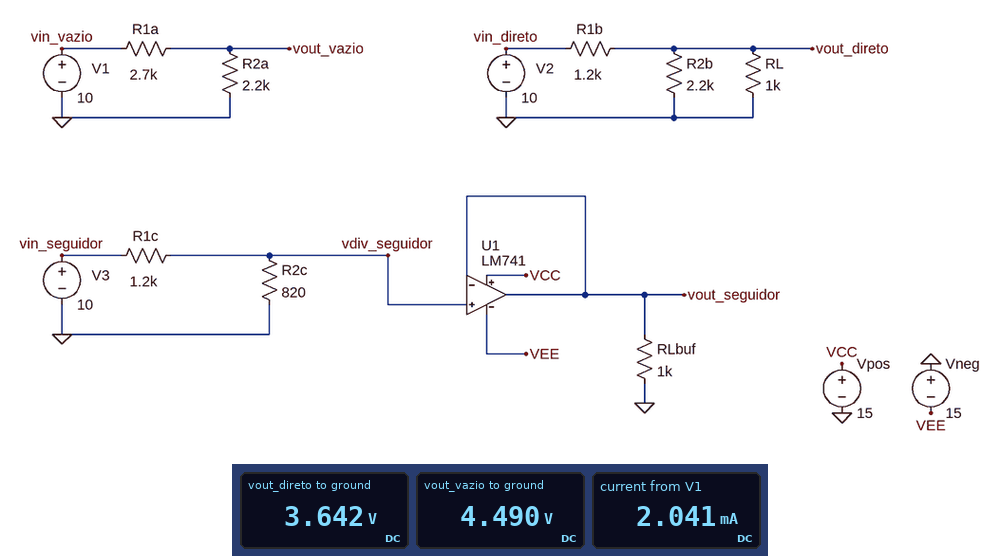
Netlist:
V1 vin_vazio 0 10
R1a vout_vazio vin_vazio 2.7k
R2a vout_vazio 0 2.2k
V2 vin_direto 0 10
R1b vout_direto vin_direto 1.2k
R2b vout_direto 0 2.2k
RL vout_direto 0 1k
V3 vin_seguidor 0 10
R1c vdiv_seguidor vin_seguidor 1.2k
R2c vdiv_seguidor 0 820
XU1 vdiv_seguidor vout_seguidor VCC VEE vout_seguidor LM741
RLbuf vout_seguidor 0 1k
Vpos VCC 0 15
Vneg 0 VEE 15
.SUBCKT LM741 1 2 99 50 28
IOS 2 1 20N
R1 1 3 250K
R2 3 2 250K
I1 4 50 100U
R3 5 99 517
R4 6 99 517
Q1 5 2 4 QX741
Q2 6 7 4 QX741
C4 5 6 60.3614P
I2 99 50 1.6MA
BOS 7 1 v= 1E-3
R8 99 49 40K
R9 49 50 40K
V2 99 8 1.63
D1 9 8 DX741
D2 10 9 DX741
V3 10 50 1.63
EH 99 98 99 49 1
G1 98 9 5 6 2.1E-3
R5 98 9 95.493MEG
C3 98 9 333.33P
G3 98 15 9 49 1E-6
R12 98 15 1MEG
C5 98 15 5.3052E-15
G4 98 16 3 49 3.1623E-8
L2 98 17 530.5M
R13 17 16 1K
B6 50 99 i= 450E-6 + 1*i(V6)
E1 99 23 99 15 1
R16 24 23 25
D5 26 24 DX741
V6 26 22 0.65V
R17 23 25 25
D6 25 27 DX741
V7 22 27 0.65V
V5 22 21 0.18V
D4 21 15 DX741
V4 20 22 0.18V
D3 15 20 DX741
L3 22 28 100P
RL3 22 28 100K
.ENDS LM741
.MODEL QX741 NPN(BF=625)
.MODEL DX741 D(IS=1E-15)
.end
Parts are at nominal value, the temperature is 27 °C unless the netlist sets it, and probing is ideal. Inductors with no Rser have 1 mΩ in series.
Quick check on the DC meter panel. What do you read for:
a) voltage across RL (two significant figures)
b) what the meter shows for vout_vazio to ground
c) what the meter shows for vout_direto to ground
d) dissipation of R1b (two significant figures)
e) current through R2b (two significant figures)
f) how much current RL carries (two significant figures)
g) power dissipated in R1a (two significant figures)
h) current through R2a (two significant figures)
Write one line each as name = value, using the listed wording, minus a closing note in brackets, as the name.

voltage across RL = 3.6 V
what the meter shows for vout_vazio to ground = 4.490 V
what the meter shows for vout_direto to ground = 3.642 V
dissipation of R1b = 34 mW
current through R2b = 1.7 mA
how much current RL carries = 3.6 mA
power dissipated in R1a = 11 mW
current through R2a = 2.0 mA
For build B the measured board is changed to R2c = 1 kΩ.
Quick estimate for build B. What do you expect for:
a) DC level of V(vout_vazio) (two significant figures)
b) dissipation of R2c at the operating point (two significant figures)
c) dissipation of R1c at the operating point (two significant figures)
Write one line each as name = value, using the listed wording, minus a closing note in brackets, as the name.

DC level of V(vout_vazio) = 4.5 V
dissipation of R2c at the operating point = 21 mW
dissipation of R1c at the operating point = 25 mW
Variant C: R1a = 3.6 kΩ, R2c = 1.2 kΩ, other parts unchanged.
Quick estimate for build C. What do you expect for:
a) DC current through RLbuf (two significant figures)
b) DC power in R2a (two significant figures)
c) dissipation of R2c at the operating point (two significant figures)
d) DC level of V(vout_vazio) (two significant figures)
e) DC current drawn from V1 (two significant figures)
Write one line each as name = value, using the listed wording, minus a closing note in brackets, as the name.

DC current through RLbuf = 5.0 mA
DC power in R2a = 6.5 mW
dissipation of R2c at the operating point = 21 mW
DC level of V(vout_vazio) = 3.8 V
DC current drawn from V1 = 1.7 mA
